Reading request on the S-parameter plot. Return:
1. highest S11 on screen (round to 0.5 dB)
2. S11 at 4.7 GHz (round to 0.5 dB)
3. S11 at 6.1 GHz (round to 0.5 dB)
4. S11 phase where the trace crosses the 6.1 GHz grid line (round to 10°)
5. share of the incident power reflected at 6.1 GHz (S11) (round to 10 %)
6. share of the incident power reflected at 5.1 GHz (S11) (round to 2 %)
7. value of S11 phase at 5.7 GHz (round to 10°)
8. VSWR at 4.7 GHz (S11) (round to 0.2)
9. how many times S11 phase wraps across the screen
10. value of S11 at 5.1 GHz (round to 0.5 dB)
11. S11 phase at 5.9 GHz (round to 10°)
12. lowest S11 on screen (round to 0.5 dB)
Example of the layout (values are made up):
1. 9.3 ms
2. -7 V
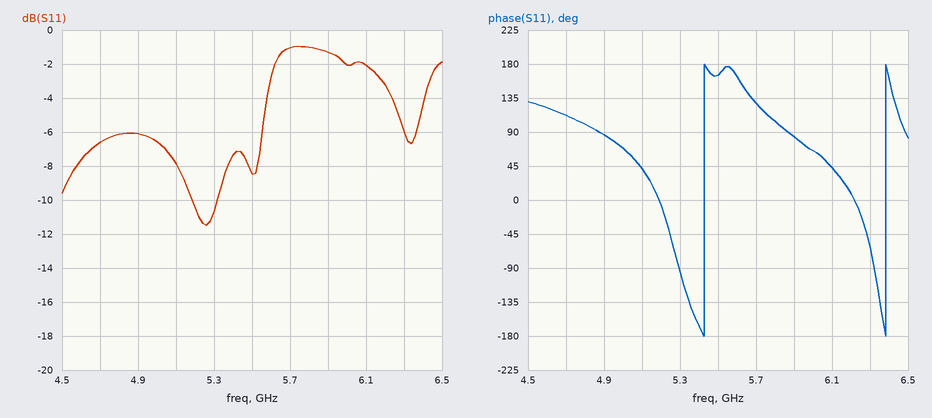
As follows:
1. -1.0 dB
2. -6.5 dB
3. -2.0 dB
4. 40°
5. 60 %
6. 16 %
7. 130°
8. 2.8
9. 2
10. -8.0 dB
11. 80°
12. -11.5 dB
